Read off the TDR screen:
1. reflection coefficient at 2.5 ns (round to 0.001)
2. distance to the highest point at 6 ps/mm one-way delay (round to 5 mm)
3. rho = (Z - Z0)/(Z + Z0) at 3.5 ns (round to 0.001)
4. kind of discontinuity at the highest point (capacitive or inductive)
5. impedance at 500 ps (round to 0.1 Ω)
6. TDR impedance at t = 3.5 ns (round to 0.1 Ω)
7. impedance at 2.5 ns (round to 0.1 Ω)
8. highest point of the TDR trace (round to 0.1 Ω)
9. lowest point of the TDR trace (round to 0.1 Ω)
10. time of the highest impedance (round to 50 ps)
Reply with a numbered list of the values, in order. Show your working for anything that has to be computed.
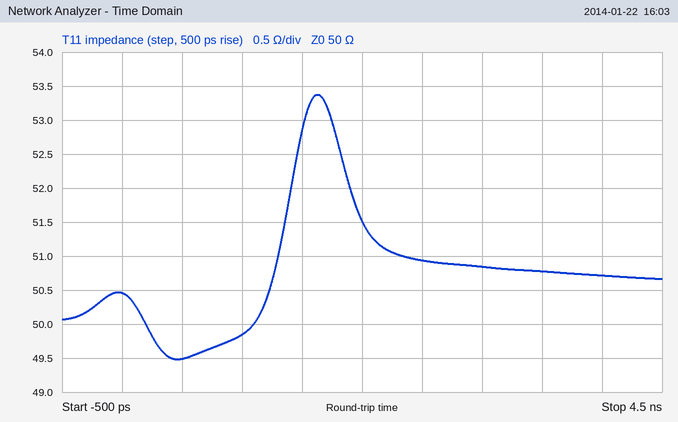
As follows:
1. (50.9 − 50)/(50.9 + 50) ≈ +0.009
2. 1.65 ns / 2 / 6 ps/mm ≈ 137 mm, so 135 mm to the nearest 5 mm
3. (50.8 − 50)/(50.8 + 50) ≈ +0.008
4. inductive
5. 49.5 Ω
6. 50.8 Ω
7. 50.9 Ω
8. 53.4 Ω
9. 49.5 Ω
10. 1.65 ns
